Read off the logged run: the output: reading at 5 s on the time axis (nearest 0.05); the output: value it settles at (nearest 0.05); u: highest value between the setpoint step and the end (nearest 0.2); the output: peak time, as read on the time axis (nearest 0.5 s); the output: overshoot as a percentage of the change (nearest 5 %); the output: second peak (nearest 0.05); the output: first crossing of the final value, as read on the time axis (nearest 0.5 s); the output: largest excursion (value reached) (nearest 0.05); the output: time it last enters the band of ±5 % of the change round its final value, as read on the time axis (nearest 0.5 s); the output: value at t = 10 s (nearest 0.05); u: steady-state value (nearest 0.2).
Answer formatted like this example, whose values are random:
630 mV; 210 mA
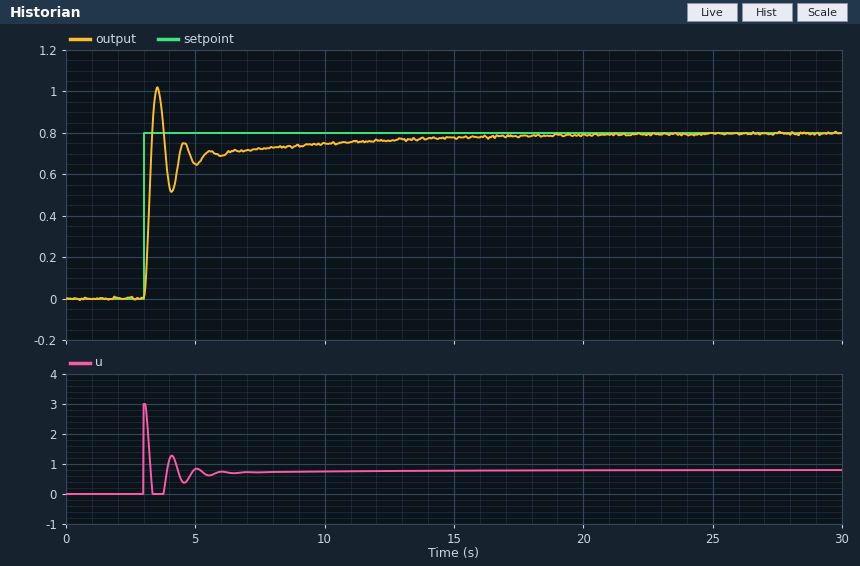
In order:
0.65; 0.80; 3.0; 3.5 s; 25 %; 0.75; 3.5 s; 1.00; 11.5 s; 0.75; 0.8
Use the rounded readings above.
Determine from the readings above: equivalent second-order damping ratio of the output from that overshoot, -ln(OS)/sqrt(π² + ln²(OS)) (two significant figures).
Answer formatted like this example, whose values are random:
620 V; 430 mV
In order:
0.40
